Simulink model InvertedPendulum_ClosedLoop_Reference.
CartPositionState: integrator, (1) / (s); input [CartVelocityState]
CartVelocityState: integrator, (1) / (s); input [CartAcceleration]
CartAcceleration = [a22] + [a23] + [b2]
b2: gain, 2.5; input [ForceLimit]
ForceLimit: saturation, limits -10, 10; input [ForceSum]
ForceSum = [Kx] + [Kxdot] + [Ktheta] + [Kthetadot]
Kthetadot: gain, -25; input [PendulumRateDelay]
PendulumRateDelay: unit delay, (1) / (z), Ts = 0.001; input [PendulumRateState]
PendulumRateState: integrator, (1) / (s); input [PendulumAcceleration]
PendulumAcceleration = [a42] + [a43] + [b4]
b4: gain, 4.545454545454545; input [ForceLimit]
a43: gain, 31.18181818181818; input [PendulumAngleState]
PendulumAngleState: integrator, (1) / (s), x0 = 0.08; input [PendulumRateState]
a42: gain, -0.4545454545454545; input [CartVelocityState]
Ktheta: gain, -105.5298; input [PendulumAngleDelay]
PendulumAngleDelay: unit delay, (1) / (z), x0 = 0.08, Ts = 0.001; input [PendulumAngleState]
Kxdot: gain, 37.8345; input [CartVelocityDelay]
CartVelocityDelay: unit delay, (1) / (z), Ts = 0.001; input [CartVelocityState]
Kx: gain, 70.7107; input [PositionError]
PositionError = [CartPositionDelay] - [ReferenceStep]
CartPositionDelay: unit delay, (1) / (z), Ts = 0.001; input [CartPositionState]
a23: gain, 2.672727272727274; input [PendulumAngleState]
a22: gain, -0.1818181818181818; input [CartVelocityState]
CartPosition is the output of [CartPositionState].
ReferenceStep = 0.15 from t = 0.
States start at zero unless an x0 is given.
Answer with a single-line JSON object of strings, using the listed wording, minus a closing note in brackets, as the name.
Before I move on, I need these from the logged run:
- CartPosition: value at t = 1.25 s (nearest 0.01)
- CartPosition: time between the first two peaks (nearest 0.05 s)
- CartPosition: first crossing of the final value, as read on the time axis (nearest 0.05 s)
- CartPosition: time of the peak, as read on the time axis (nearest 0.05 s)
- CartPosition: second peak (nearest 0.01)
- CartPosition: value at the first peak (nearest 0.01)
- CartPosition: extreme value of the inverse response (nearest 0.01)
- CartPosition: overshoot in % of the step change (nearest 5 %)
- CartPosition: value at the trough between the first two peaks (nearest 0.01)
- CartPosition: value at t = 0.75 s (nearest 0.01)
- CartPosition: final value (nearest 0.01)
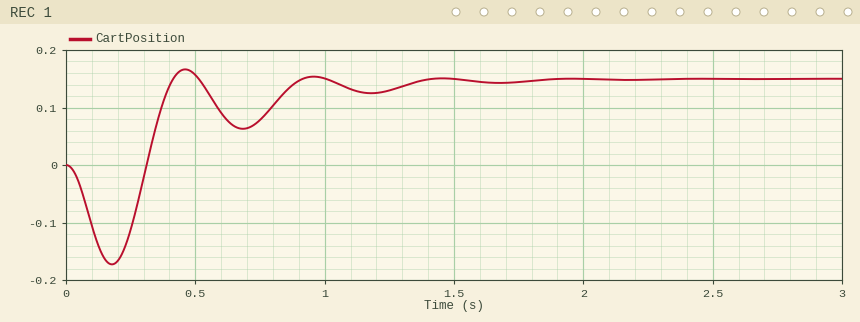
{"CartPosition: value at t = 1.25 s": "0.13", "CartPosition: time between the first two peaks": "0.50 s", "CartPosition: first crossing of the final value, as read on the time axis": "0.40 s", "CartPosition: time of the peak, as read on the time axis": "0.45 s", "CartPosition: second peak": "0.15", "CartPosition: value at the first peak": "0.17", "CartPosition: extreme value of the inverse response": "-0.17", "CartPosition: overshoot in % of the step change": "10 %", "CartPosition: value at the trough between the first two peaks": "0.06", "CartPosition: value at t = 0.75 s": "0.08", "CartPosition: final value": "0.15"}
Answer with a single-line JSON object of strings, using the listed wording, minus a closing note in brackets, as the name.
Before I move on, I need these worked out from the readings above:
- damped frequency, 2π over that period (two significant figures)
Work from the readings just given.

{"damped frequency, 2π over that period": "13 rad/s"}
